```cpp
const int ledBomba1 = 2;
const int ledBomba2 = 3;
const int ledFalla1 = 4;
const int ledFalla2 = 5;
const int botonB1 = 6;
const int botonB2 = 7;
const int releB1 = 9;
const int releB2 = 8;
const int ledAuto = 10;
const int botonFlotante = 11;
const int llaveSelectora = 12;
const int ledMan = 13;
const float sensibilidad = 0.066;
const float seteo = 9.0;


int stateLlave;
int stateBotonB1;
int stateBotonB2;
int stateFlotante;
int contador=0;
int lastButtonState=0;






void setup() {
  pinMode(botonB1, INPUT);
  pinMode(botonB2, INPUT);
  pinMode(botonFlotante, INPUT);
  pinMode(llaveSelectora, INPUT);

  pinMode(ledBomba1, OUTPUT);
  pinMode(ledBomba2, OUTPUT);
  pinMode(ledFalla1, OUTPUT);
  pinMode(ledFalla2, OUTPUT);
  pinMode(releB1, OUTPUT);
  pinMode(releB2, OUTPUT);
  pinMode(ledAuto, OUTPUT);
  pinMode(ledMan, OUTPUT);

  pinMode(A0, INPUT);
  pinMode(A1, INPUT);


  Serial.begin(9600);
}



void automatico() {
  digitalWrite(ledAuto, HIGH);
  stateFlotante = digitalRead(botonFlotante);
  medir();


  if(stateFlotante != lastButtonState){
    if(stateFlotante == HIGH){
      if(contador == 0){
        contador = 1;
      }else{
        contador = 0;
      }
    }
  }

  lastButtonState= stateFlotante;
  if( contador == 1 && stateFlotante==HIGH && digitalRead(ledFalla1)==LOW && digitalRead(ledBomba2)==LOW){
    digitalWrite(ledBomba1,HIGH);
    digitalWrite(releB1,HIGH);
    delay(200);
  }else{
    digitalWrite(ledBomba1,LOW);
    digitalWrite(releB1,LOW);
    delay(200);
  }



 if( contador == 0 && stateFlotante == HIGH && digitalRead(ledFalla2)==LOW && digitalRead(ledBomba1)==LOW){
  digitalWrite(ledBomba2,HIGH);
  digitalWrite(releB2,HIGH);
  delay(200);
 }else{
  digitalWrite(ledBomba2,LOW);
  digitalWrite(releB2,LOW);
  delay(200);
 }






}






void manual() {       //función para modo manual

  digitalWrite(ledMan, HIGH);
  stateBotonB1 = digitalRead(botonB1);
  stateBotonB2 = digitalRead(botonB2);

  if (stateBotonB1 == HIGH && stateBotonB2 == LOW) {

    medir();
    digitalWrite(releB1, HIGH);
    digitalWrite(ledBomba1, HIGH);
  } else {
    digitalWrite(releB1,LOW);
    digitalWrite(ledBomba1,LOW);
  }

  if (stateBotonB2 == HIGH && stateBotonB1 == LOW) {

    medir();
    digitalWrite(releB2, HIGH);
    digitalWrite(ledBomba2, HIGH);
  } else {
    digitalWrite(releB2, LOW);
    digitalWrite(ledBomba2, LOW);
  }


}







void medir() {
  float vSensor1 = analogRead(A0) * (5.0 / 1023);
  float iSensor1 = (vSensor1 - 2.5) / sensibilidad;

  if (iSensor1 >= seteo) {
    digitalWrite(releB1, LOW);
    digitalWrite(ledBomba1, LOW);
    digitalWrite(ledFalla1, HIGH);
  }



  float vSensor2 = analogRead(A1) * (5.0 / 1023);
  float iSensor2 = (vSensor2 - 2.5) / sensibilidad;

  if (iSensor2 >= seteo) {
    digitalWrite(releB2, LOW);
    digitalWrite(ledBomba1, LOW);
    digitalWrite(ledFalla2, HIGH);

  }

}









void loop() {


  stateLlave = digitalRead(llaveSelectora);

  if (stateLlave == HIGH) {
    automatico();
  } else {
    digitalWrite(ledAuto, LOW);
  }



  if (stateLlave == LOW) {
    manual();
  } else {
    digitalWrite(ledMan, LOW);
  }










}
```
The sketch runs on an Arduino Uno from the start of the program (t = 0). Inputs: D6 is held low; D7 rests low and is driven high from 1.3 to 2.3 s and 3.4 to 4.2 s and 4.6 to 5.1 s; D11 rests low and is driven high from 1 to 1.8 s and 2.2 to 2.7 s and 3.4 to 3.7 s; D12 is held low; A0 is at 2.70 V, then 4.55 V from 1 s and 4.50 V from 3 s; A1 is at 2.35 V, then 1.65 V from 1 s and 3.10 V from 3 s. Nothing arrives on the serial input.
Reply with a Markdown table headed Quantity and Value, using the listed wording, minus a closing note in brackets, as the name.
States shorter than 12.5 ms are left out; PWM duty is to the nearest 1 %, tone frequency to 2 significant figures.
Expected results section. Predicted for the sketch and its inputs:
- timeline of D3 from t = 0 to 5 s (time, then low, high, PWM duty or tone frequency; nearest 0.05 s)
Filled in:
| Quantity | Value |
|---|---|
| timeline of D3 from t = 0 to 5 s | 0 s low; 1.3 s high; 2.3 s low; 3.4 s high; 4.2 s low; 4.6 s high |
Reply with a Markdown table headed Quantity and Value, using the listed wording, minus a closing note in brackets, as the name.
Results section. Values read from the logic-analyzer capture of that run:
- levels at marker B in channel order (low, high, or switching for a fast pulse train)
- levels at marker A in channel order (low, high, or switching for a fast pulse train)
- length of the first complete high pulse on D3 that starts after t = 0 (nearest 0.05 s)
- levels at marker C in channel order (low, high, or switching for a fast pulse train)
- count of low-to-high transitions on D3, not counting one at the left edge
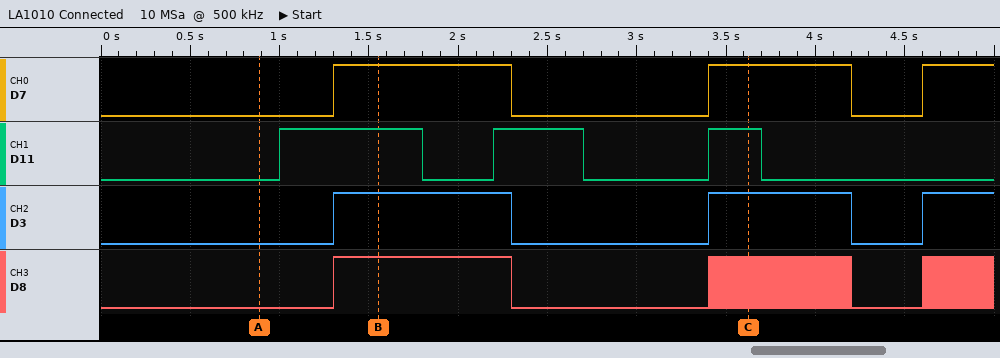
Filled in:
| Quantity | Value |
|---|---|
| levels at marker B in channel order | D7 high, D11 high, D3 high, D8 high |
| levels at marker A in channel order | D7 low, D11 low, D3 low, D8 low |
| length of the first complete high pulse on D3 that starts after t = 0 | 1.00 s |
| levels at marker C in channel order | D7 high, D11 high, D3 high, D8 switching |
| count of low-to-high transitions on D3, not counting one at the left edge | 3 |
